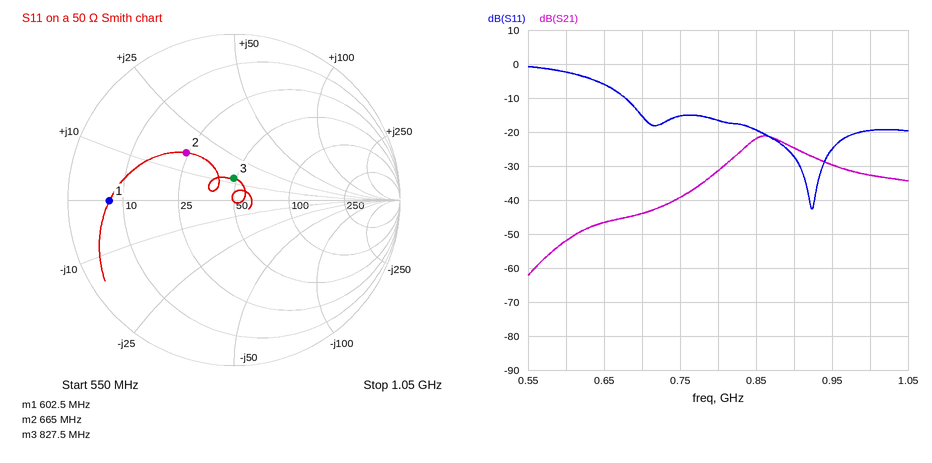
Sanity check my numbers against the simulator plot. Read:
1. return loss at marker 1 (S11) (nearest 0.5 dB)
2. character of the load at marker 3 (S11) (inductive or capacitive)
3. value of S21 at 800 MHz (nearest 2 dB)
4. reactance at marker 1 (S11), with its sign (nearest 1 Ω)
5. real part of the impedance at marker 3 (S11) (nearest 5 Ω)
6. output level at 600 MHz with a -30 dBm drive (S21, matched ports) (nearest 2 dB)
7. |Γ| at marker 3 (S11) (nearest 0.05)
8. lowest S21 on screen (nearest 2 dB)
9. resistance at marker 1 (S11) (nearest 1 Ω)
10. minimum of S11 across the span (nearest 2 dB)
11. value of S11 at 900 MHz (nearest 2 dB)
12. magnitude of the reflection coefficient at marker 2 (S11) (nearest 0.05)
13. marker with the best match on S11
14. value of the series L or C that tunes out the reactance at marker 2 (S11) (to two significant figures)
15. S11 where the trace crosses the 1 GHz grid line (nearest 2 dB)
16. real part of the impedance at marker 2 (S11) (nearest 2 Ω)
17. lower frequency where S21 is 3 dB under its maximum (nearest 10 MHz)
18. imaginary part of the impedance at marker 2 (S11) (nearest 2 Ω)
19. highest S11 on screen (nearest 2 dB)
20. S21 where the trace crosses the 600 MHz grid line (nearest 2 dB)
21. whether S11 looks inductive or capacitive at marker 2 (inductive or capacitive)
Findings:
2.5 dB
inductive
-32 dB
0 Ω
50 Ω
-82 dBm
0.15
-62 dB
7 Ω
-42 dB
-28 dB
0.40
marker 3
15 pF
-20 dB
24 Ω
840 MHz
+16 Ω
0 dB
-52 dB
inductive
